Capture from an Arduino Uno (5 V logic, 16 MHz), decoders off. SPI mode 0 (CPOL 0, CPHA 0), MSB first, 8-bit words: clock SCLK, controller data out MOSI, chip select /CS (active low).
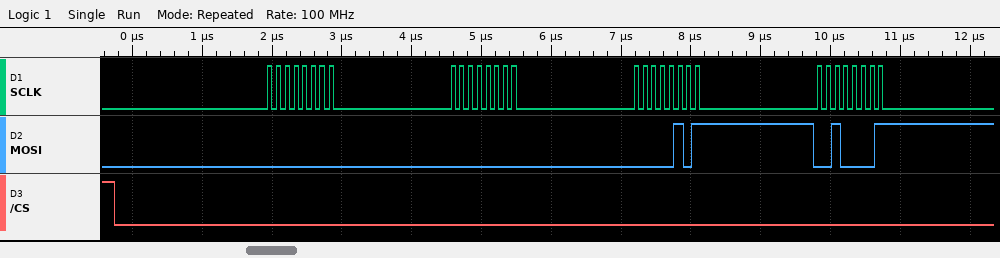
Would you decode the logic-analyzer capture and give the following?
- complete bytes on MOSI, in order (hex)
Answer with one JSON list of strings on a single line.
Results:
["00 00 05 21"]
